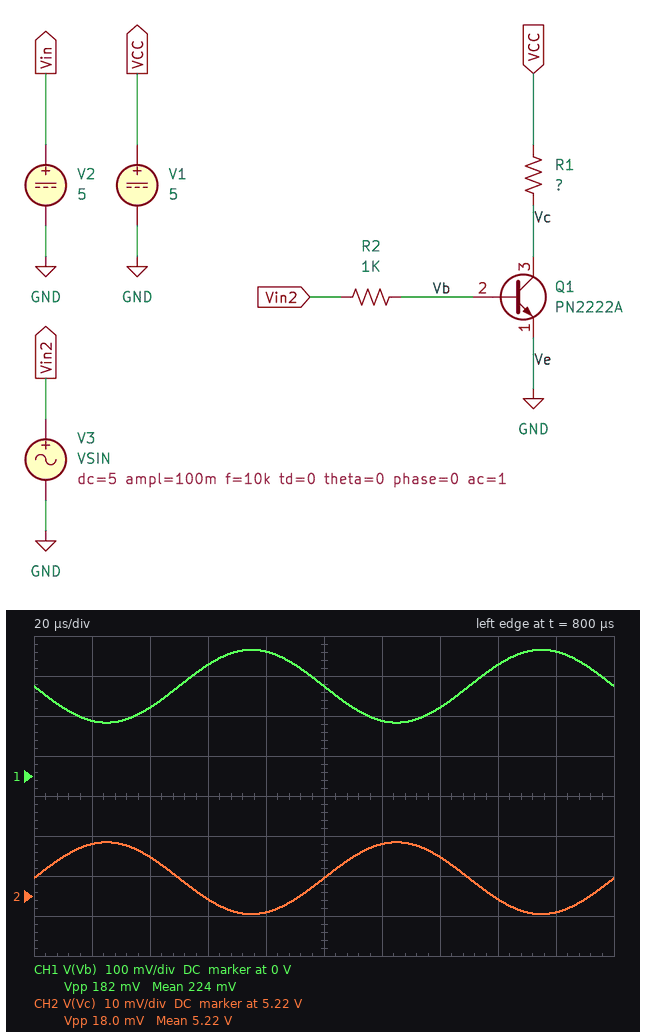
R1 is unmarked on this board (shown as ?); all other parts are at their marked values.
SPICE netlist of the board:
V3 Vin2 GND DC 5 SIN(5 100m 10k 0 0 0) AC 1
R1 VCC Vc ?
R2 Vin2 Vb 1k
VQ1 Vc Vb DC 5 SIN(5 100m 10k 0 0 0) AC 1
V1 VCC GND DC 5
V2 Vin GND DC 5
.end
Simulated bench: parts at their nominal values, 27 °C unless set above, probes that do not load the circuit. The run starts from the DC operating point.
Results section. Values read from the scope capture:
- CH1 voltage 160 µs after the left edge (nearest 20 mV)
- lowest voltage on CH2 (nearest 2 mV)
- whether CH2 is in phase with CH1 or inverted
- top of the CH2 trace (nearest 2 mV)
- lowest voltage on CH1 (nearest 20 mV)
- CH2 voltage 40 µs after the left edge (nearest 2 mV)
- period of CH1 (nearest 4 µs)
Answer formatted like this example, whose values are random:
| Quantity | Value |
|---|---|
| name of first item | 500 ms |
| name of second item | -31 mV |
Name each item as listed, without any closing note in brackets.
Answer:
| Quantity | Value |
|---|---|
| CH1 voltage 160 µs after the left edge | 280 mV |
| lowest voltage on CH2 | 5.216 V |
| whether CH2 is in phase with CH1 or inverted | inverted |
| top of the CH2 trace | 5.234 V |
| lowest voltage on CH1 | 140 mV |
| CH2 voltage 40 µs after the left edge | 5.230 V |
| period of CH1 | 100 µs |
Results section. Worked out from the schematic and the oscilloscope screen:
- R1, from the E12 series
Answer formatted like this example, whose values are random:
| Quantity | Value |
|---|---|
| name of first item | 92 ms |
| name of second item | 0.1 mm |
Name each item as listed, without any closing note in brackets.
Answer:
| Quantity | Value |
|---|---|
| R1, from the E12 series | 47 Ω |
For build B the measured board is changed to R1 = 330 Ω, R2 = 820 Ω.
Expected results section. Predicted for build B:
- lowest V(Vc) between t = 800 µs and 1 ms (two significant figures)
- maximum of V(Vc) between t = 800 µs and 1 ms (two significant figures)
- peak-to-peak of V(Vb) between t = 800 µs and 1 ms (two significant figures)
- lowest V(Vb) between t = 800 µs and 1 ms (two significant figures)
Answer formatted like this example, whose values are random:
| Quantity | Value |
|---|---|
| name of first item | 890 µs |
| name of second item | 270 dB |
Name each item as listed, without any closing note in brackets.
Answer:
| Quantity | Value |
|---|---|
| lowest V(Vc) between t = 800 µs and 1 ms | 6.4 V |
| maximum of V(Vc) between t = 800 µs and 1 ms | 6.5 V |
| peak-to-peak of V(Vb) between t = 800 µs and 1 ms | 85 mV |
| lowest V(Vb) between t = 800 µs and 1 ms | 1.4 V |
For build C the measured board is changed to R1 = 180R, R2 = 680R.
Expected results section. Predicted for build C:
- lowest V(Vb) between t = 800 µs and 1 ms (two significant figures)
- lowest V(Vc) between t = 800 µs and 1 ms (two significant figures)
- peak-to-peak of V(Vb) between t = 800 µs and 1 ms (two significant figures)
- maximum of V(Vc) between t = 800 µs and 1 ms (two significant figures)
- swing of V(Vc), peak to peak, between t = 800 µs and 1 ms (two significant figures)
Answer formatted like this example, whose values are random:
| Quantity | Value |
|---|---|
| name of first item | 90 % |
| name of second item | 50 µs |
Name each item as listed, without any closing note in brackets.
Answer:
| Quantity | Value |
|---|---|
| lowest V(Vb) between t = 800 µs and 1 ms | 990 mV |
| lowest V(Vc) between t = 800 µs and 1 ms | 6.0 V |
| peak-to-peak of V(Vb) between t = 800 µs and 1 ms | 120 mV |
| maximum of V(Vc) between t = 800 µs and 1 ms | 6.1 V |
| swing of V(Vc), peak to peak, between t = 800 µs and 1 ms | 84 mV |
